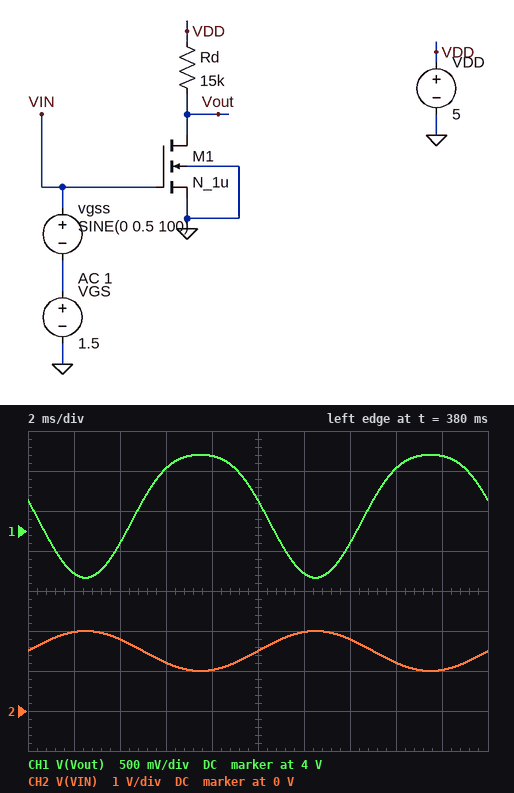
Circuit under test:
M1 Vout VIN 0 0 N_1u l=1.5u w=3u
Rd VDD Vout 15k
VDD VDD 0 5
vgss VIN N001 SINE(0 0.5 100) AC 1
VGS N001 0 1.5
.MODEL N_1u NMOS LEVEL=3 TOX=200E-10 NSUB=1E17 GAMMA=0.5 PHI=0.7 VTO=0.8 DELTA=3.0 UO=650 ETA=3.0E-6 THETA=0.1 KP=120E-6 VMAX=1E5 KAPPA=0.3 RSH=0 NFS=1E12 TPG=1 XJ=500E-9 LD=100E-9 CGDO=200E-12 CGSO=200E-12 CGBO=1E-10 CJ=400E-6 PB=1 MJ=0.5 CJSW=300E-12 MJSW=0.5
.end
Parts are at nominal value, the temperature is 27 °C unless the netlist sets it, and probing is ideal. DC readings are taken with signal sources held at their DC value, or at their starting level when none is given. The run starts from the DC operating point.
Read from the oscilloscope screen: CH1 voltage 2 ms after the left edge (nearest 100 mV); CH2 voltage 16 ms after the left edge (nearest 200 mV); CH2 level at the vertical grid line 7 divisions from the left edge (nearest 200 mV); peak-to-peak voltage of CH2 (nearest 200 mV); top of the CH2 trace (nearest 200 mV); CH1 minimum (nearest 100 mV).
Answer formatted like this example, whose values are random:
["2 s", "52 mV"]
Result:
["3.5 V", "1.2 V", "1.8 V", "1.0 V", "2.0 V", "3.4 V"]
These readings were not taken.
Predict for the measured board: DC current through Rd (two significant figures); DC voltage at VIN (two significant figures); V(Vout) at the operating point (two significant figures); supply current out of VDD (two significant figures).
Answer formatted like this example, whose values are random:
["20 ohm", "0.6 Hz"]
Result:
["41 µA", "1.5 V", "4.4 V", "41 µA"]
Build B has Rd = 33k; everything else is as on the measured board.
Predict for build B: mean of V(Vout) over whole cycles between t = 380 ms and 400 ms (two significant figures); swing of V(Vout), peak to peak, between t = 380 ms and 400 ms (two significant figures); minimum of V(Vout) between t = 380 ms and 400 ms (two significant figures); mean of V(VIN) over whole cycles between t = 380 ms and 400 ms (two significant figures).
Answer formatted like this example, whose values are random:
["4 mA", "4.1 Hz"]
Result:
["3.5 V", "3.3 V", "1.6 V", "1.5 V"]
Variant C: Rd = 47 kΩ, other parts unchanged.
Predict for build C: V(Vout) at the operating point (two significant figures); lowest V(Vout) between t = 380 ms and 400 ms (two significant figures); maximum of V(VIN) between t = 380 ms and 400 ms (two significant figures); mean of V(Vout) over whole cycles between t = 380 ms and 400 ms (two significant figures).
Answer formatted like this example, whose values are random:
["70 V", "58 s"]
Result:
["3.1 V", "600 mV", "2.0 V", "2.9 V"]
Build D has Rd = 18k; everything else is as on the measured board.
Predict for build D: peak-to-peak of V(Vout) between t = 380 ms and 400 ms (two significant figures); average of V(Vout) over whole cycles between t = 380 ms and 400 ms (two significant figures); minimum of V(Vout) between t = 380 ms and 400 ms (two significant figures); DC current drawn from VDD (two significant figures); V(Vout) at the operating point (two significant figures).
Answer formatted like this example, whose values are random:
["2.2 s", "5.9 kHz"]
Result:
["1.8 V", "4.1 V", "3.1 V", "41 µA", "4.3 V"]
